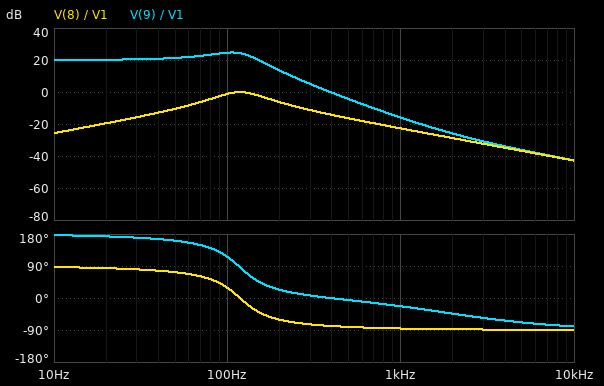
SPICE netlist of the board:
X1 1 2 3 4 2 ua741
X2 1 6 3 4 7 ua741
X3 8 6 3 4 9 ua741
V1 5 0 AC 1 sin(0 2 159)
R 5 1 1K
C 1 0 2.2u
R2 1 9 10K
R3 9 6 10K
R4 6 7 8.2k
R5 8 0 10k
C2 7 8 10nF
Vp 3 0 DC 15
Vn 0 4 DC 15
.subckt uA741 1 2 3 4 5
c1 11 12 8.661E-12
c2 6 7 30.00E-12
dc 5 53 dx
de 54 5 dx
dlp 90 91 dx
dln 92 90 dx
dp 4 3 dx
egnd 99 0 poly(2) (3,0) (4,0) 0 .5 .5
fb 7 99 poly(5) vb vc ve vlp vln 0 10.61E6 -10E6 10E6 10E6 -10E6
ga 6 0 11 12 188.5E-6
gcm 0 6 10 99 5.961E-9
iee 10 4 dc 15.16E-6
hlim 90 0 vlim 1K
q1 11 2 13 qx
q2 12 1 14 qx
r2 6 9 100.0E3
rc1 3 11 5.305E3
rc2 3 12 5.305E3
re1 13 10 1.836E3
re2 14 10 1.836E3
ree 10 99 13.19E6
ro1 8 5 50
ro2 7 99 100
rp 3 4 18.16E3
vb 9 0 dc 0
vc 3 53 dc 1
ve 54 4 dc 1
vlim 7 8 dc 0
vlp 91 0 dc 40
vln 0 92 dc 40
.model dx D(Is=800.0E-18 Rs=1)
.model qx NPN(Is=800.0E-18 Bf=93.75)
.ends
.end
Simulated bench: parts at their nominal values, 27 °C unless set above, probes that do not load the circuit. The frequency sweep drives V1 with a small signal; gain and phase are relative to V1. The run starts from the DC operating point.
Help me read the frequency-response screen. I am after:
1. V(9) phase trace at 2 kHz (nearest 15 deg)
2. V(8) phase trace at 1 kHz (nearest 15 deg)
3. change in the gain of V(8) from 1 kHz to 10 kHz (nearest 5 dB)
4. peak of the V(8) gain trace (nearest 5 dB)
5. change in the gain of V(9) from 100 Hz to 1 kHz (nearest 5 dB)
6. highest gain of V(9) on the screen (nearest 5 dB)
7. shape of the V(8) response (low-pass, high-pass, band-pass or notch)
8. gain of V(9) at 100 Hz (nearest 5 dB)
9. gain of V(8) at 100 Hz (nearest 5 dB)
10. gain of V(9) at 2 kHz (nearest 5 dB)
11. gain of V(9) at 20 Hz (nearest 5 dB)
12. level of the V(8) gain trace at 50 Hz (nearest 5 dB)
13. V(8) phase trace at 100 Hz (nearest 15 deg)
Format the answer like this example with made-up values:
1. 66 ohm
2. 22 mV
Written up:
1. -45 deg
2. -90 deg
3. -20 dB
4. 0 dB
5. -40 dB
6. 25 dB
7. band-pass
8. 25 dB
9. 0 dB
10. -25 dB
11. 20 dB
12. -10 dB
13. 30 deg
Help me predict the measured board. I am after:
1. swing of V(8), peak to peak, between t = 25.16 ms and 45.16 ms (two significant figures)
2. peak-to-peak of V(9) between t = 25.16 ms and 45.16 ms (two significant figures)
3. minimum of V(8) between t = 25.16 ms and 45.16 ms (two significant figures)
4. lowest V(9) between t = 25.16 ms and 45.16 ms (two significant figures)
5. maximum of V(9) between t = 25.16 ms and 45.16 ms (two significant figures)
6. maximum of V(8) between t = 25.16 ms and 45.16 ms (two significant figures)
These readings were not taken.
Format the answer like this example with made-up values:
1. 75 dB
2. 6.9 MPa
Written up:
1. 2.6 V
2. 29 V
3. -1.3 V
4. -15 V
5. 15 V
6. 1.3 V
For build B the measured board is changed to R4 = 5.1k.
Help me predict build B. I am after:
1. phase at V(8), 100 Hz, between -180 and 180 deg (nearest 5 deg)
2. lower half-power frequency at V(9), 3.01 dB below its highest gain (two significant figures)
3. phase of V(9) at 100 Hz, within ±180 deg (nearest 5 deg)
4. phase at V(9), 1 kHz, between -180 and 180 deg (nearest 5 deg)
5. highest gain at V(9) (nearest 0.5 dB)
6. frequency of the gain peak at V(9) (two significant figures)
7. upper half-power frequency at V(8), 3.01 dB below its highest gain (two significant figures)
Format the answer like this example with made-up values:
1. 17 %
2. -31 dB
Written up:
1. 60 deg
2. 97 Hz
3. 150 deg
4. -15 deg
5. 26.5 dB
6. 140 Hz
7. 190 Hz
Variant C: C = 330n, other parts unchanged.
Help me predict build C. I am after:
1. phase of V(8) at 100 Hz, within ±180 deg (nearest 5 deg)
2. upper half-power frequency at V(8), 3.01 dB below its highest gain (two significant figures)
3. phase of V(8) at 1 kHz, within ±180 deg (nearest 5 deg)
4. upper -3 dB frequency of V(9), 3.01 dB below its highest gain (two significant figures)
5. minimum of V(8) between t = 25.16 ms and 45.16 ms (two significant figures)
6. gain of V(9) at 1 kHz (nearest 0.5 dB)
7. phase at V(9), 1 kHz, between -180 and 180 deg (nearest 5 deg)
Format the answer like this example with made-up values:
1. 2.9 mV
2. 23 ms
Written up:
1. 60 deg
2. 630 Hz
3. -60 deg
4. 270 Hz
5. -1.4 V
6. 0 dB
7. 0 deg
